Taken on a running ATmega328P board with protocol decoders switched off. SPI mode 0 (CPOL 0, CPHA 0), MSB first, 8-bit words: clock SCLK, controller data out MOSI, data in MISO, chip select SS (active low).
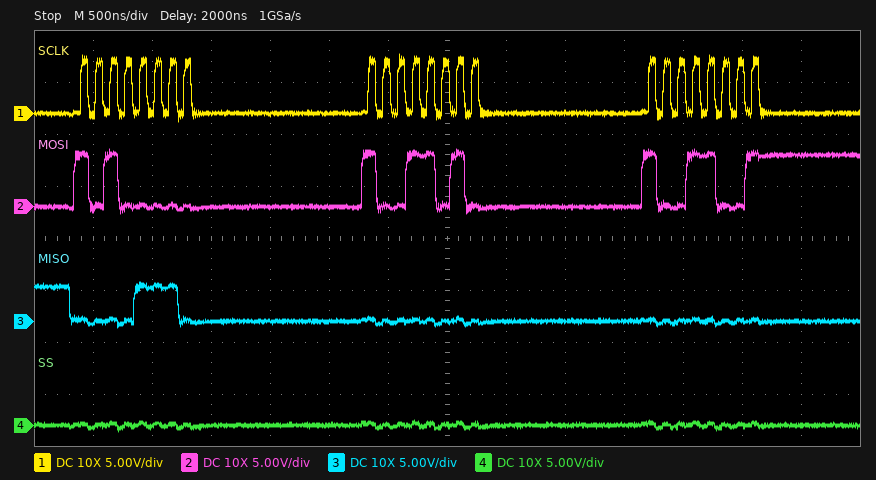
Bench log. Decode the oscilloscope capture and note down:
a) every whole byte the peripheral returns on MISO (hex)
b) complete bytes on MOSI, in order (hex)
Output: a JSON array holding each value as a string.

["0E 00 00", "A0 9A 99"]
